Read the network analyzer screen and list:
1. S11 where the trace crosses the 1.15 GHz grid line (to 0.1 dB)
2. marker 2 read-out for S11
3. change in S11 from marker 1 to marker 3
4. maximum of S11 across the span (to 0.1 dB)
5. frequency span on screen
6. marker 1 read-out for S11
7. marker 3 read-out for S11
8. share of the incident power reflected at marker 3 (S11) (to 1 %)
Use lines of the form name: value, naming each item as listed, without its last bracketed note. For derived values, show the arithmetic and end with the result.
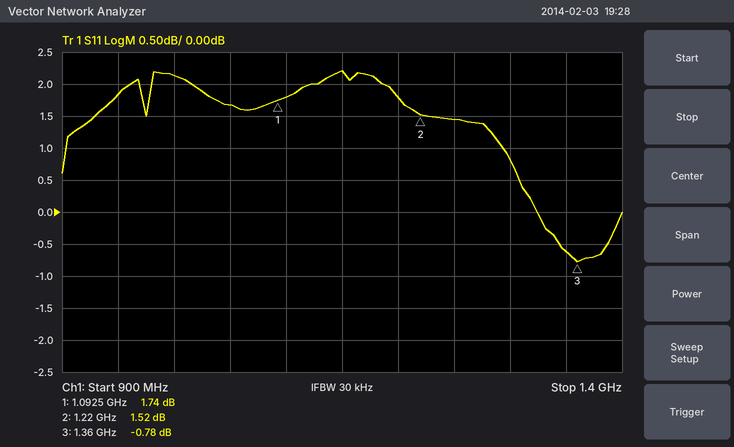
S11 where the trace crosses the 1.15 GHz grid line: 2.2 dB
marker 2 read-out for S11: 1.52 dB
change in S11 from marker 1 to marker 3: -0.78 − (1.74) = -2.52 dB
maximum of S11 across the span: 2.2 dB
frequency span on screen: 500 MHz
marker 1 read-out for S11: 1.74 dB
marker 3 read-out for S11: -0.78 dB
share of the incident power reflected at marker 3 (S11): 10^(-0.78/10) ≈ 84 %
